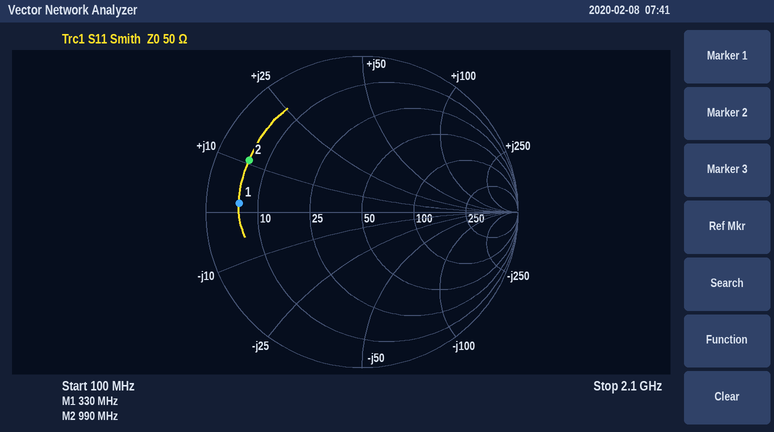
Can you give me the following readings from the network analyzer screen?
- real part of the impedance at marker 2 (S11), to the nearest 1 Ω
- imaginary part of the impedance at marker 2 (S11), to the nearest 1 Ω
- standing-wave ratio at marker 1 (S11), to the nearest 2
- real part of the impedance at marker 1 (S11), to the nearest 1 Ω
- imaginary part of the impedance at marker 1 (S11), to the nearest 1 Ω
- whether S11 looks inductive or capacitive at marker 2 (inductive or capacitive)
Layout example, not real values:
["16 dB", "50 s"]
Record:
["6 Ω", "+11 Ω", "8", "6 Ω", "+2 Ω", "inductive"]
